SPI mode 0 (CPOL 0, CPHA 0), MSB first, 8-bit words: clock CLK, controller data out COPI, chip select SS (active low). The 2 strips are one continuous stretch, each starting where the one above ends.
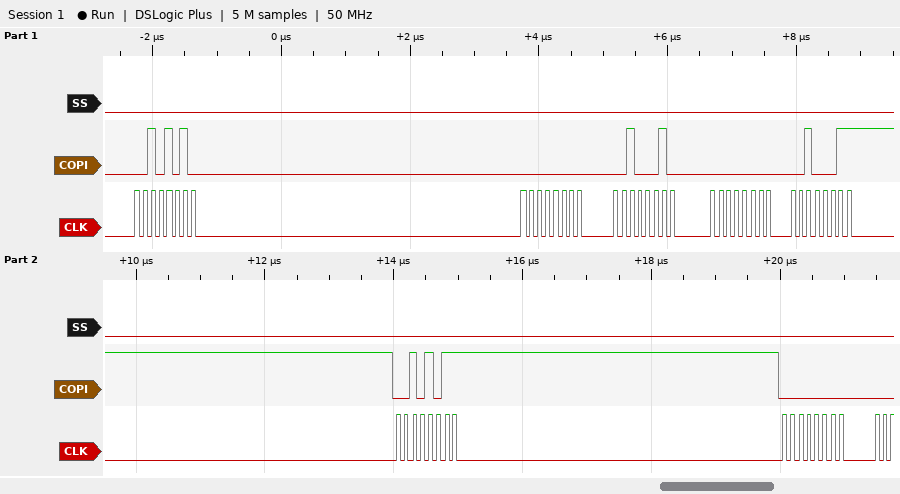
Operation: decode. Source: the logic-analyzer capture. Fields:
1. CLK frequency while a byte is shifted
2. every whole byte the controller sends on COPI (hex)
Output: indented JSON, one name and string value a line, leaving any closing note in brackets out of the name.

{
  "CLK frequency while a byte is shifted": "8 MHz",
  "every whole byte the controller sends on COPI": "2A 00 22 00 23 2B 00"
}
